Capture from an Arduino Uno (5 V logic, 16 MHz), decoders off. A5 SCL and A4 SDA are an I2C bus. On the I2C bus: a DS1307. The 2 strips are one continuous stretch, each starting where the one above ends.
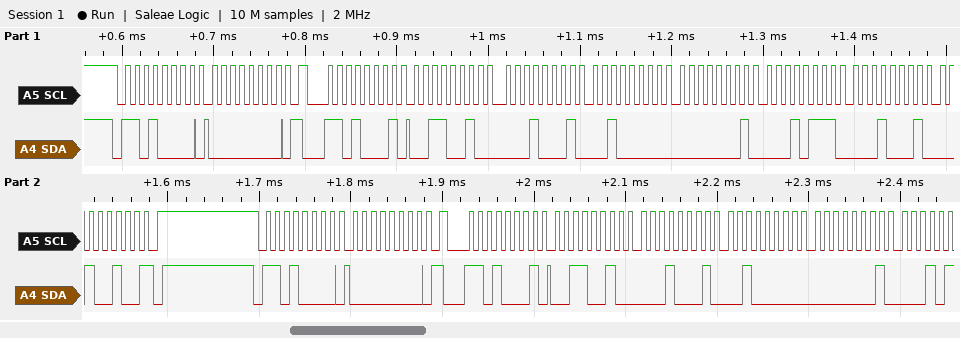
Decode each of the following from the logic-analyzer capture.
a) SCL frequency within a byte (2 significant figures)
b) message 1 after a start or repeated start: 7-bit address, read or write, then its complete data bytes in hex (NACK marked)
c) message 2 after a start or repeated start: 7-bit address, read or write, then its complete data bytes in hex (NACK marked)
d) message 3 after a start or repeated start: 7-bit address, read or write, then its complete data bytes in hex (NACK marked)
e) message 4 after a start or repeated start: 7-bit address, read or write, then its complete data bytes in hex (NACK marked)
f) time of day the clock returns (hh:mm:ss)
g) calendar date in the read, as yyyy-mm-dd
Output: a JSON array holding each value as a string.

["100 kHz", "0x68 write: 00", "0x68 read: 32 11 20 01 17 11 24 NACK", "0x68 write: 00", "0x68 read: 32 11 20 01", "20:11:32", "2024-11-17"]
